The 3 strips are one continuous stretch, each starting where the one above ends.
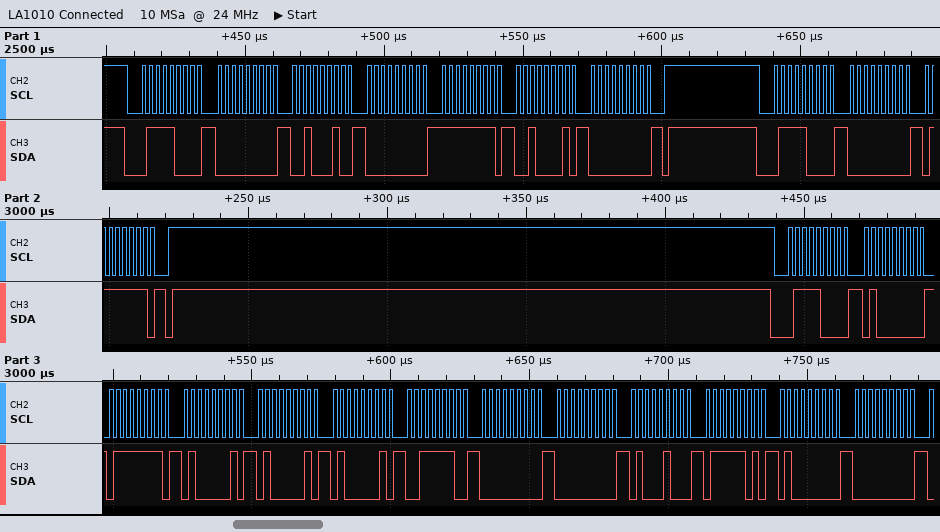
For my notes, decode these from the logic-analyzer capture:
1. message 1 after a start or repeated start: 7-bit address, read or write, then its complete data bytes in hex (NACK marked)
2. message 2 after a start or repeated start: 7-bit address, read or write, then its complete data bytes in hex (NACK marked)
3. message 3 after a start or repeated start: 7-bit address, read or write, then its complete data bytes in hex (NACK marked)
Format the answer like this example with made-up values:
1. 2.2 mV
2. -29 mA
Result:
1. 0x3C write: 00 22 00 FF 21 00
2. 0x3C write: 00 7F
3. 0x3C write: 40 7F 41 41 41 3E 00 00 44 7D 40 00
